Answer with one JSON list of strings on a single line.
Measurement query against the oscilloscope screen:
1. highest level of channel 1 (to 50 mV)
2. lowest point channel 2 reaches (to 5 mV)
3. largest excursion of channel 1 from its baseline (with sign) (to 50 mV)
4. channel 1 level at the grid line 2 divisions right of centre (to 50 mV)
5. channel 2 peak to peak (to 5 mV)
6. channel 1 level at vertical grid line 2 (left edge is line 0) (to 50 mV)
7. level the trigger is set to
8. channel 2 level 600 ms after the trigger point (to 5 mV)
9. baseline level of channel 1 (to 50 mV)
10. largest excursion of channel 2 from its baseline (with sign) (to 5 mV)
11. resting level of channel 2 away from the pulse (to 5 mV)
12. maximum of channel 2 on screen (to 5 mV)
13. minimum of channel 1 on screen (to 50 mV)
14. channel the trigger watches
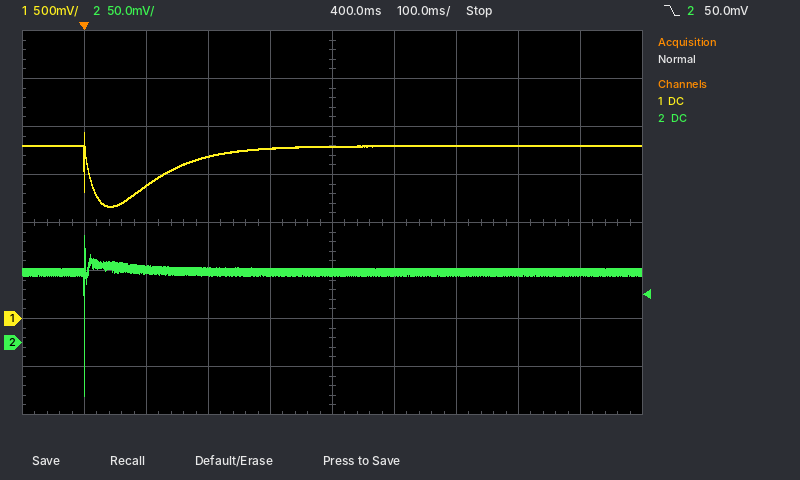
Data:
["1.95 V", "-55 mV", "-650 mV", "1.80 V", "165 mV", "1.40 V", "50.0 mV", "75 mV", "1.80 V", "-130 mV", "75 mV", "110 mV", "1.15 V", "channel 2"]
